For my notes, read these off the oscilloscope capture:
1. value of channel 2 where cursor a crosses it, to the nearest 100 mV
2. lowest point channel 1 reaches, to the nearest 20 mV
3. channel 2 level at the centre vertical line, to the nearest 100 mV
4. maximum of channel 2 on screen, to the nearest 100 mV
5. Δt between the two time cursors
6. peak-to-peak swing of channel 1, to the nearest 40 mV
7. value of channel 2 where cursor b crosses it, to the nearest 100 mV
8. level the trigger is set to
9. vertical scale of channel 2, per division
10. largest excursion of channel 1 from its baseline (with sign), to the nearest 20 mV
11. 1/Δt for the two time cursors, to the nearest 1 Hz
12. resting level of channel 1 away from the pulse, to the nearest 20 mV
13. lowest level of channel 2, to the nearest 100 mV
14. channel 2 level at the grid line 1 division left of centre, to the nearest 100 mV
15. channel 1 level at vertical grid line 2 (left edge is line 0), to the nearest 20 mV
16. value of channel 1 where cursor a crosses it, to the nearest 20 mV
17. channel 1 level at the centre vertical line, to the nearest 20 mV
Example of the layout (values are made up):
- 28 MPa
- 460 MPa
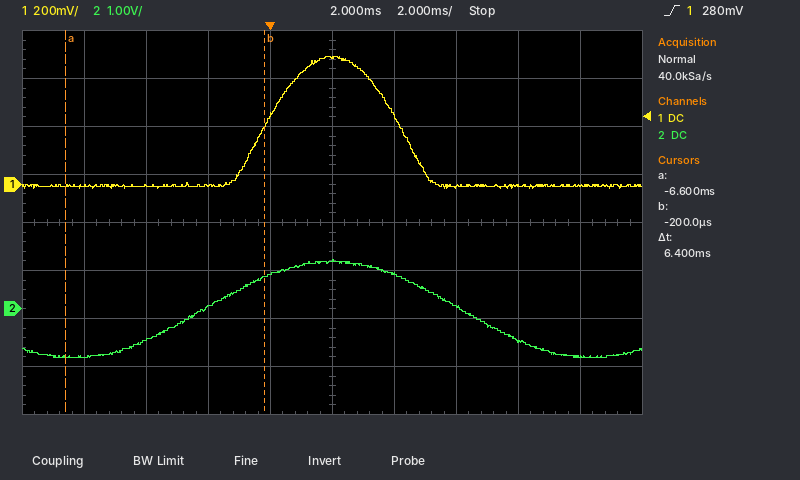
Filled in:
- -1.0 V
- -20 mV
- 1.0 V
- 1.0 V
- 6.4 ms
- 560 mV
- 700 mV
- 280 mV
- 1 V
- +540 mV
- 156 Hz
- 0 mV
- -1.0 V
- 700 mV
- 0 mV
- 0 mV
- 520 mV
